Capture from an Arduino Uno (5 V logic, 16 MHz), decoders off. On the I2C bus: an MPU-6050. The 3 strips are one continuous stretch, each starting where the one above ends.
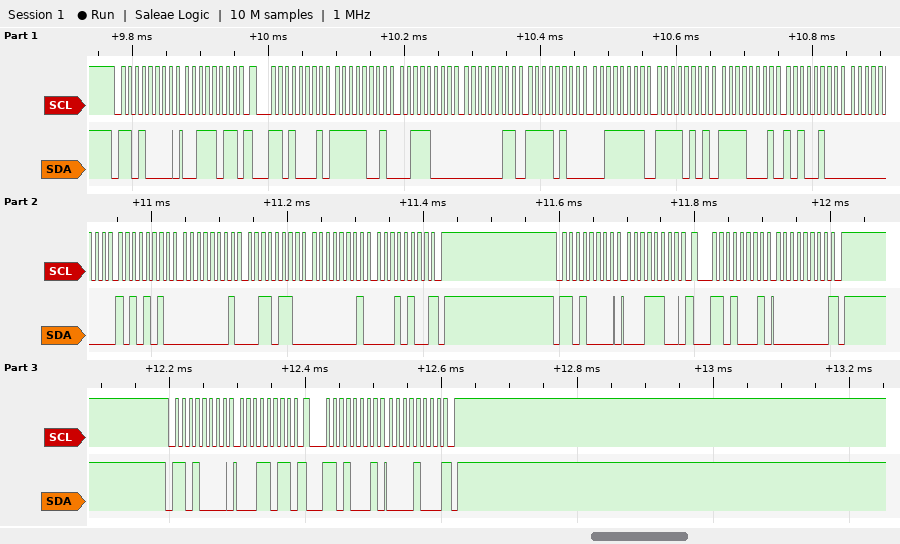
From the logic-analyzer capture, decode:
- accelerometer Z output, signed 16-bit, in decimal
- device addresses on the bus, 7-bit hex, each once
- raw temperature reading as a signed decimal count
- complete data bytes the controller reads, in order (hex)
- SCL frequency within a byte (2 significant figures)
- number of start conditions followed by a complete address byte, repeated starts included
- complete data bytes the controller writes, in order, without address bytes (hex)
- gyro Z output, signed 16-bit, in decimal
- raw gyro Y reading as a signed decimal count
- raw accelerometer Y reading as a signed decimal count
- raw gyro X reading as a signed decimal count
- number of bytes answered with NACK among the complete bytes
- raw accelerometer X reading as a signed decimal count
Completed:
16373
0x68
-3676
F9 38 03 F4 3F F5 F1 A4 00 AA 01 36 01 14 00 08
100 kHz
6
3B 1C 1B
276
310
1012
170
3
-1736
